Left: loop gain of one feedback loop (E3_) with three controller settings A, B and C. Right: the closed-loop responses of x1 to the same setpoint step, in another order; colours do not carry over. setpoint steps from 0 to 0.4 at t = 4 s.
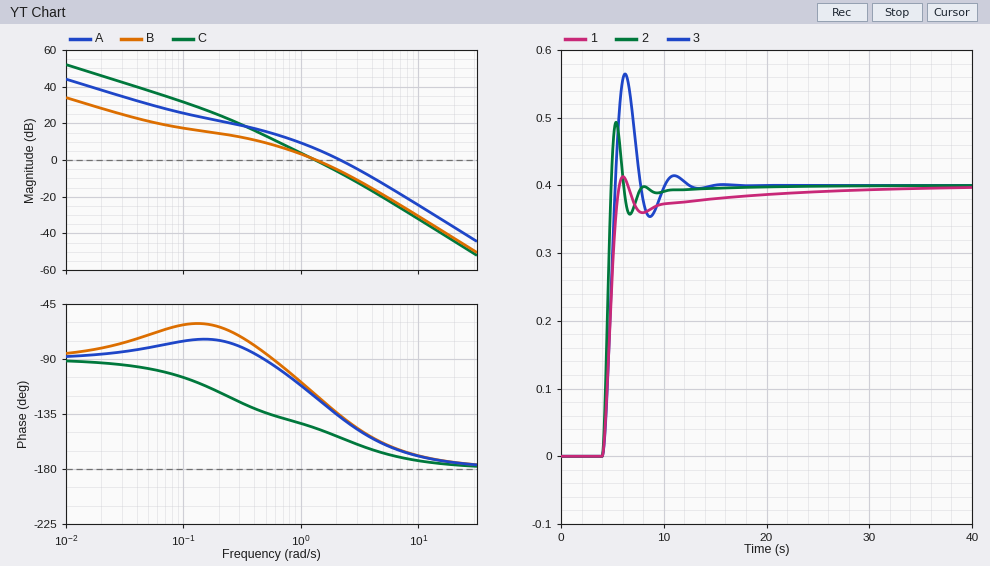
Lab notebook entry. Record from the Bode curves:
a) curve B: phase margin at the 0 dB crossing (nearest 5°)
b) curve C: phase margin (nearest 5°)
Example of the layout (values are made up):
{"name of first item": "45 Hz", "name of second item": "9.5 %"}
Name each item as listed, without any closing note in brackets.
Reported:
{"curve B: phase margin at the 0 dB crossing": "60°", "curve C: phase margin": "35°"}
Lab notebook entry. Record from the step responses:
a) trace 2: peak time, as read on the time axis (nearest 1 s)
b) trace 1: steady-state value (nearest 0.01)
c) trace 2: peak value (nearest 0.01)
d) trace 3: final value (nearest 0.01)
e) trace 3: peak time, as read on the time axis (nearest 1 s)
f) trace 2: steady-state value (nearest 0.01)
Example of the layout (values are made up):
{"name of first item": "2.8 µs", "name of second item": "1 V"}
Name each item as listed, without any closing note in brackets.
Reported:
{"trace 2: peak time, as read on the time axis": "5 s", "trace 1: steady-state value": "0.40", "trace 2: peak value": "0.49", "trace 3: final value": "0.40", "trace 3: peak time, as read on the time axis": "6 s", "trace 2: steady-state value": "0.40"}
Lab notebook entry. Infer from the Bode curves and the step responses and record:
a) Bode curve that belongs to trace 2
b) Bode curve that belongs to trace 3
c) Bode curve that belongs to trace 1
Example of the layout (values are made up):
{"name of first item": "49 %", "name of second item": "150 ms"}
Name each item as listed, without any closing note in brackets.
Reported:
{"Bode curve that belongs to trace 2": "A", "Bode curve that belongs to trace 3": "C", "Bode curve that belongs to trace 1": "B"}
